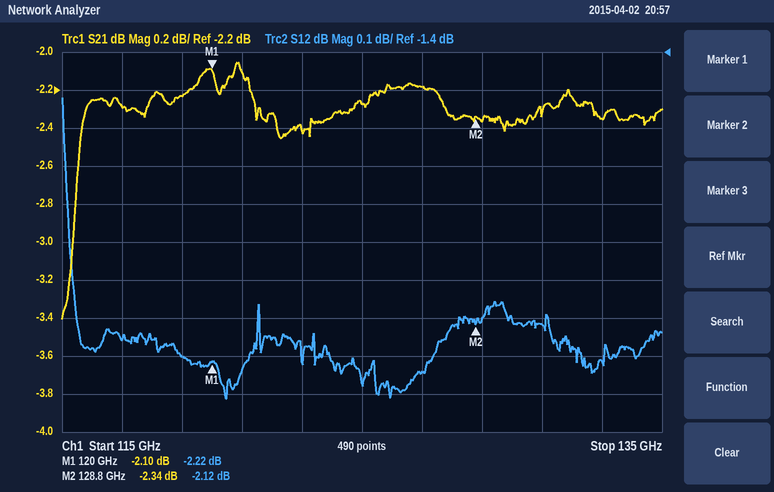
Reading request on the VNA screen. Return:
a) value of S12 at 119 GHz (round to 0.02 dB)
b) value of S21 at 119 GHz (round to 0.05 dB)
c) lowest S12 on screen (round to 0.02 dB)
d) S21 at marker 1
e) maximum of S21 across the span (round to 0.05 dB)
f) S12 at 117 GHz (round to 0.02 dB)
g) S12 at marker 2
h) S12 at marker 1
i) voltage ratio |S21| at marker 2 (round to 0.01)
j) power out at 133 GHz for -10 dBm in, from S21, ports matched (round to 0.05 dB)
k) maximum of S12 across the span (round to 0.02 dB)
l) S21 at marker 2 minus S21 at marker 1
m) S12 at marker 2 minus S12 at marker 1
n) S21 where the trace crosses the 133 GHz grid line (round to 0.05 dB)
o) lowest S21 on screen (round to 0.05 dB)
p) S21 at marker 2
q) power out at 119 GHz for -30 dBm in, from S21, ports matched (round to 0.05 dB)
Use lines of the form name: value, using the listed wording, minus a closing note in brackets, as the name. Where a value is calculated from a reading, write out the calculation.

value of S12 at 119 GHz: -2.20 dB
value of S21 at 119 GHz: -2.25 dB
lowest S12 on screen: -2.32 dB
S21 at marker 1: -2.10 dB
maximum of S21 across the span: -2.05 dB
S12 at 117 GHz: -2.16 dB
S12 at marker 2: -2.12 dB
S12 at marker 1: -2.22 dB
voltage ratio |S21| at marker 2: 10^(-2.34/20) ≈ 0.76
power out at 133 GHz for -10 dBm in, from S21, ports matched: -10 dBm + (-2.35 dB) = -12.35 dBm
maximum of S12 across the span: -1.52 dB
S21 at marker 2 minus S21 at marker 1: -2.34 − (-2.1) = -0.24 dB
S12 at marker 2 minus S12 at marker 1: -2.12 − (-2.22) = 0.10 dB
S21 where the trace crosses the 133 GHz grid line: -2.35 dB
lowest S21 on screen: -3.40 dB
S21 at marker 2: -2.34 dB
power out at 119 GHz for -30 dBm in, from S21, ports matched: -30 dBm + (-2.25 dB) = -32.25 dBm
